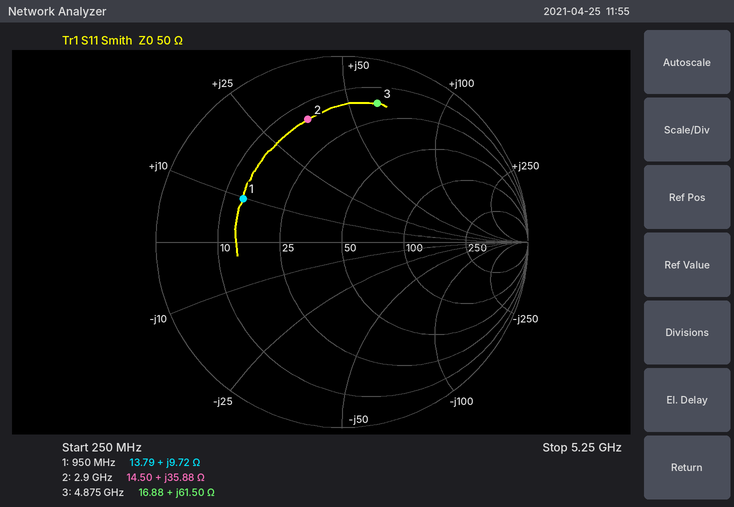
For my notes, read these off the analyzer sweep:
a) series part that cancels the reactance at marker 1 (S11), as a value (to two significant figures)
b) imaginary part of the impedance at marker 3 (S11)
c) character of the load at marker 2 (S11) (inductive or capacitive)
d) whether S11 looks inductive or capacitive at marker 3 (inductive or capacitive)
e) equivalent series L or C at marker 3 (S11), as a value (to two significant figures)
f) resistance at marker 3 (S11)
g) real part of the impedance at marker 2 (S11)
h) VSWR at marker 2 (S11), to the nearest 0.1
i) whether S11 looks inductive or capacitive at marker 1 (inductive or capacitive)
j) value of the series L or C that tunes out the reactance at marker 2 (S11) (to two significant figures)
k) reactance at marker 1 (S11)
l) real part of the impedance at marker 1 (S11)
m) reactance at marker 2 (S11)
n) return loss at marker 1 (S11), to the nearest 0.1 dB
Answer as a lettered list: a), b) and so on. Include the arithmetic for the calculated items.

a) C = 1/(2π × 950 MHz × 9.72 Ω) ≈ 17 pF
b) +61.50 Ω
c) inductive
d) inductive
e) L = 61.5 Ω/(2π × 4.875 GHz) ≈ 2.0 nH
f) 16.88 Ω
g) 14.50 Ω
h) 5.3
i) inductive
j) C = 1/(2π × 2.9 GHz × 35.88 Ω) ≈ 1.5 pF
k) +9.72 Ω
l) 13.79 Ω
m) +35.88 Ω
n) 4.7 dB
